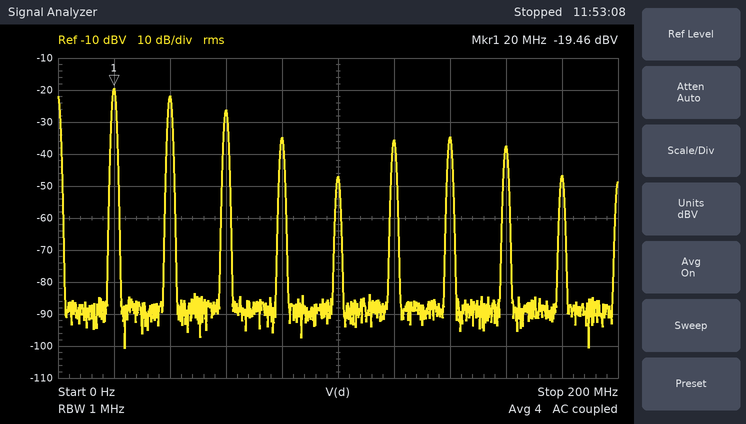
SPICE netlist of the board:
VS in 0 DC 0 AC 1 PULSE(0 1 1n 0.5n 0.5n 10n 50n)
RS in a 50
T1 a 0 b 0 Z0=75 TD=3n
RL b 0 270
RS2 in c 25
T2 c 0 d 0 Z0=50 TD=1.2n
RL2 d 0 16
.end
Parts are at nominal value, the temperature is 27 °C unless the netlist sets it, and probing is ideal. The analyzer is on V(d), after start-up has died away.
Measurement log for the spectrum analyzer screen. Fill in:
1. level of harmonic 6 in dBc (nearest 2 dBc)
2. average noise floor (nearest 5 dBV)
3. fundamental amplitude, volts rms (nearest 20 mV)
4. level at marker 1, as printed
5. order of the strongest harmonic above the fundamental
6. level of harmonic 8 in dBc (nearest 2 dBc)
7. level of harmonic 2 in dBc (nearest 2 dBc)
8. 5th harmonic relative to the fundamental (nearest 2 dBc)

-16 dBc
-90 dBV
100 mV
-19.46 dBV
2
-18 dBc
-2 dBc
-28 dBc
